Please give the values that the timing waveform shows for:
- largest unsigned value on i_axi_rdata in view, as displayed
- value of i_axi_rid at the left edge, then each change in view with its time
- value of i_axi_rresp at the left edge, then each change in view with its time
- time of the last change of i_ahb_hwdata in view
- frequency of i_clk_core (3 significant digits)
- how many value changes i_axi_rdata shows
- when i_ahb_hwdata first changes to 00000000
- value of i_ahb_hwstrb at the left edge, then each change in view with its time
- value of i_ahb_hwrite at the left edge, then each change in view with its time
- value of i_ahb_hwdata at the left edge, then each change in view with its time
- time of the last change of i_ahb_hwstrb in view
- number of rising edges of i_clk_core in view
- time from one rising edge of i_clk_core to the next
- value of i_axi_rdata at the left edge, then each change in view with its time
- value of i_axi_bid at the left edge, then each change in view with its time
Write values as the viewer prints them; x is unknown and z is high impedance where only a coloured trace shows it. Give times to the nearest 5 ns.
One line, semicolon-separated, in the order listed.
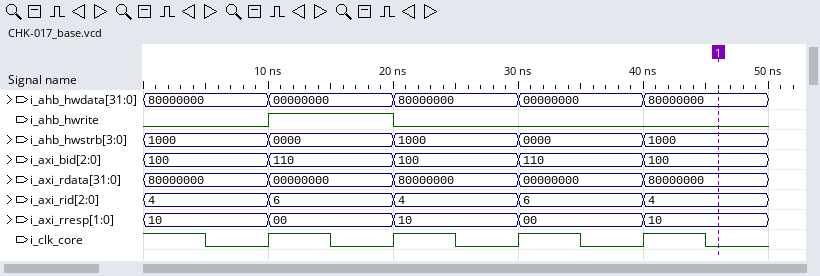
80000000; 4, 6 at 10 ns, 4 at 20 ns, 6 at 30 ns, 4 at 40 ns; 10, 00 at 10 ns, 10 at 20 ns, 00 at 30 ns, 10 at 40 ns; 40 ns; 100 MHz; 4; 10 ns; 1000, 0000 at 10 ns, 1000 at 20 ns, 0000 at 30 ns, 1000 at 40 ns; 0, 1 at 10 ns, 0 at 20 ns; 80000000, 00000000 at 10 ns, 80000000 at 20 ns, 00000000 at 30 ns, 80000000 at 40 ns; 40 ns; 4; 10 ns; 80000000, 00000000 at 10 ns, 80000000 at 20 ns, 00000000 at 30 ns, 80000000 at 40 ns; 100, 110 at 10 ns, 100 at 20 ns, 110 at 30 ns, 100 at 40 ns
